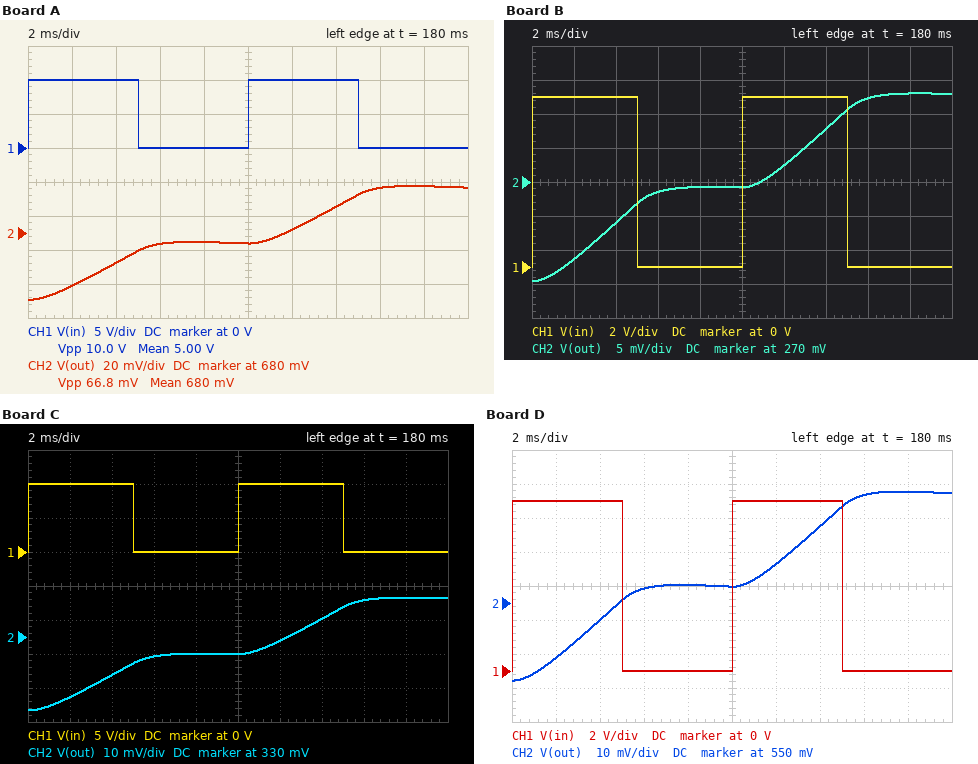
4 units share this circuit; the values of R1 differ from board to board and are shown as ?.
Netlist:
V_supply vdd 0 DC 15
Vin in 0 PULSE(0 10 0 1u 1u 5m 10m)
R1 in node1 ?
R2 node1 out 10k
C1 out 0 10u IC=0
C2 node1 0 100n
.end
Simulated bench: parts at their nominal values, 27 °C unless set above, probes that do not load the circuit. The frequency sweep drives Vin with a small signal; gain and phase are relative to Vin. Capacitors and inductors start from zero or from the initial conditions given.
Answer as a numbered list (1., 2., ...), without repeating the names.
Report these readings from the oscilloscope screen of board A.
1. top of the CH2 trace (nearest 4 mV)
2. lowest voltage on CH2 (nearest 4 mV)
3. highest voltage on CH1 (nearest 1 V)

1. 708 mV
2. 640 mV
3. 10 V
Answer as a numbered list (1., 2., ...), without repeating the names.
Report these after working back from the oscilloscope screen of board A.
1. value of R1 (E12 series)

1. 120 kΩ
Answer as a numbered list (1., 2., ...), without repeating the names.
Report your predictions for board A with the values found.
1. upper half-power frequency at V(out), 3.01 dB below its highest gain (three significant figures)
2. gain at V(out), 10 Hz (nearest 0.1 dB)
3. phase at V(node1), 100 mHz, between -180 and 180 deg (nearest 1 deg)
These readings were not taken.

1. 121 mHz
2. -38.3 dB
3. -36 deg
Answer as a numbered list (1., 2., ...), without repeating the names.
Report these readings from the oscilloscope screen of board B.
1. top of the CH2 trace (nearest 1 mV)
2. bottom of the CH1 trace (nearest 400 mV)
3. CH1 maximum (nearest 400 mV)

1. 283 mV
2. 0 V
3. 10.0 V
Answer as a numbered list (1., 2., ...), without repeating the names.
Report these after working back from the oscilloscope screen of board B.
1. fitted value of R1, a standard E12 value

1. 330 kΩ
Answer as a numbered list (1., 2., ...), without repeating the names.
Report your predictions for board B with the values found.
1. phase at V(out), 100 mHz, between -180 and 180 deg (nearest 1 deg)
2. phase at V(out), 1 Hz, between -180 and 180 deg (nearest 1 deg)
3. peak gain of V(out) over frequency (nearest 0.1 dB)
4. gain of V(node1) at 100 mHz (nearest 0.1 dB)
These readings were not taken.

1. -65 deg
2. -88 deg
3. 0 dB
4. -7.5 dB
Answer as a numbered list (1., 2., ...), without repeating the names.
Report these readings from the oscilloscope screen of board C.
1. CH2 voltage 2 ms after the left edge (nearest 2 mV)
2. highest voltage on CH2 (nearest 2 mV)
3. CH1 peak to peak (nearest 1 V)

1. 312 mV
2. 342 mV
3. 10 V
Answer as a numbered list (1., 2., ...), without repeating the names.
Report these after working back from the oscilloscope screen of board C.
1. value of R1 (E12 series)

1. 270 kΩ
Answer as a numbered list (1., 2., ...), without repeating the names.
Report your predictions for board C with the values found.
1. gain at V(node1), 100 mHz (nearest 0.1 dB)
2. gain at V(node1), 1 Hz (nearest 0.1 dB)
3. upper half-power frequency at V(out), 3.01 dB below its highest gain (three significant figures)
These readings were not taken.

1. -6.2 dB
2. -23.6 dB
3. 56.3 mHz
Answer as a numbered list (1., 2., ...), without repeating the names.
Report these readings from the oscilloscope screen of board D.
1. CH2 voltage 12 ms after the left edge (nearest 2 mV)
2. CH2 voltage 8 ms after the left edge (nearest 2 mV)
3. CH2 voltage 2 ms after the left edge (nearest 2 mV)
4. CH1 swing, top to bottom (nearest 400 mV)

1. 562 mV
2. 556 mV
3. 534 mV
4. 10.0 V
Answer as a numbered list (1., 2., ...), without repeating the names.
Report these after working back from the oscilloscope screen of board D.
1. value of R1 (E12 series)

1. 150 kΩ
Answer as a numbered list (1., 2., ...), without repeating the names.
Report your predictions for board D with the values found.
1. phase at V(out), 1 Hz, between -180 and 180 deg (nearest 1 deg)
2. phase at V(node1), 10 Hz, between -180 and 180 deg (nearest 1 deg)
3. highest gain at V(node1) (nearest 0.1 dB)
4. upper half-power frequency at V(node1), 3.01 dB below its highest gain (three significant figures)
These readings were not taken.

1. -85 deg
2. -12 deg
3. 0 dB
4. 99.0 mHz
